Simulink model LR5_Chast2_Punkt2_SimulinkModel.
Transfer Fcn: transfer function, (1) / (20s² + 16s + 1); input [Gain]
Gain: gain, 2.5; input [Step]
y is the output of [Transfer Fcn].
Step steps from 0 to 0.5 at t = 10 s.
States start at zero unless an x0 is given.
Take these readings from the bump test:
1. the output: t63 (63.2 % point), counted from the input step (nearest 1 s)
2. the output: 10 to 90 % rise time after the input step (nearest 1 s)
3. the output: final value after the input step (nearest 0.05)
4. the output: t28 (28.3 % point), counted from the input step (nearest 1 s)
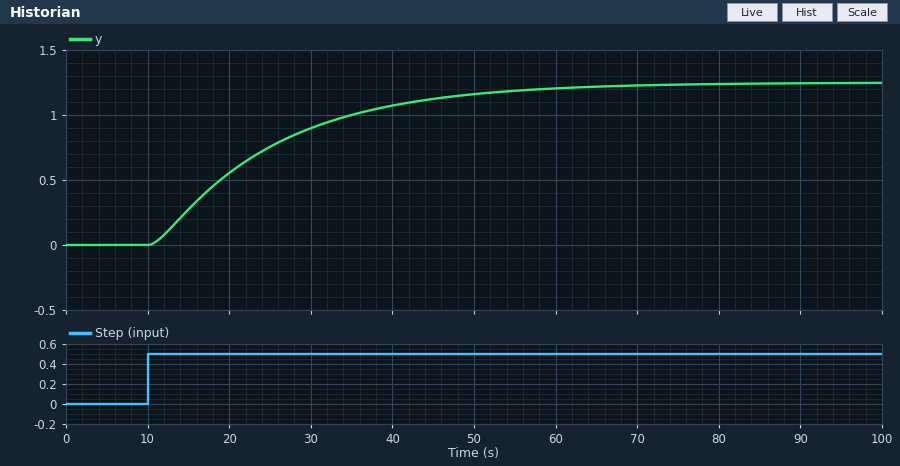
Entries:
16 s
32 s
1.25
6 s
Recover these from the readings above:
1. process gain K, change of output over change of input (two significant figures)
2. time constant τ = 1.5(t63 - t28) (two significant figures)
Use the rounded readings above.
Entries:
2.5
15 s
